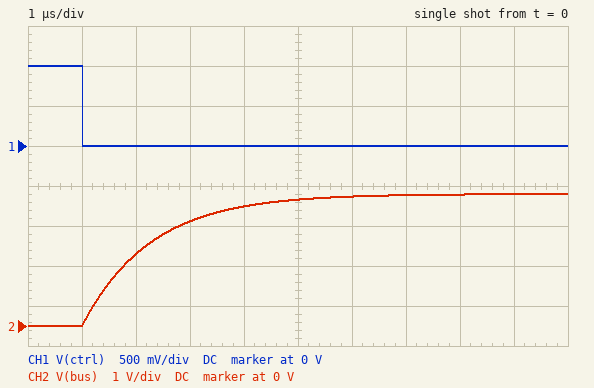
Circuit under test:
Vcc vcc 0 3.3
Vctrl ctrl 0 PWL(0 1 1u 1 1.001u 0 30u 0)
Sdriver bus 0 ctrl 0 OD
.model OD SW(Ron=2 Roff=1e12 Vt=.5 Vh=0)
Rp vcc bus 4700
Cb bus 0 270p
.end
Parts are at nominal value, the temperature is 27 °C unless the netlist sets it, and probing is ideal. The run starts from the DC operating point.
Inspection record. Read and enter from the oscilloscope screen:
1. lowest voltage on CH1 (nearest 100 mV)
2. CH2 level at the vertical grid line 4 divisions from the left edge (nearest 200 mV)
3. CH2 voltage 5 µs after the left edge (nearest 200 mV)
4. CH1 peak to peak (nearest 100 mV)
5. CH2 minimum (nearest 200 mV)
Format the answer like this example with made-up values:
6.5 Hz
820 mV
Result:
0 V
3.0 V
3.2 V
1.0 V
0 V
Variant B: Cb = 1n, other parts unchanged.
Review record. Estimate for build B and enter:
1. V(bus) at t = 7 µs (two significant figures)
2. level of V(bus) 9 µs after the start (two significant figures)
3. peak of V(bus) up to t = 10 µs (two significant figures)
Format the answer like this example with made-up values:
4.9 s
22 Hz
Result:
2.4 V
2.7 V
2.8 V
